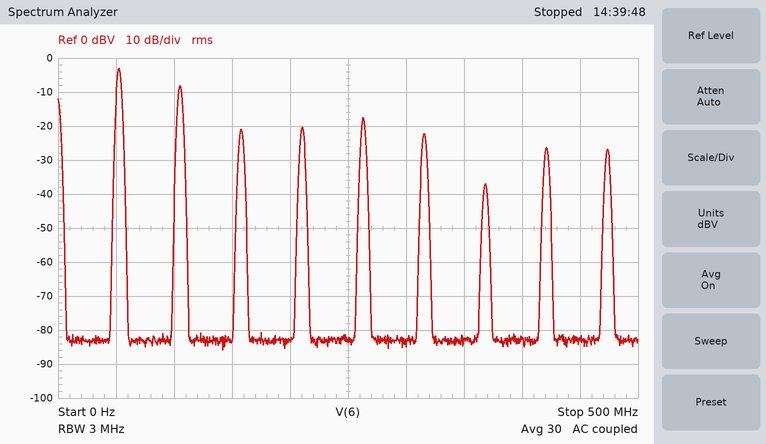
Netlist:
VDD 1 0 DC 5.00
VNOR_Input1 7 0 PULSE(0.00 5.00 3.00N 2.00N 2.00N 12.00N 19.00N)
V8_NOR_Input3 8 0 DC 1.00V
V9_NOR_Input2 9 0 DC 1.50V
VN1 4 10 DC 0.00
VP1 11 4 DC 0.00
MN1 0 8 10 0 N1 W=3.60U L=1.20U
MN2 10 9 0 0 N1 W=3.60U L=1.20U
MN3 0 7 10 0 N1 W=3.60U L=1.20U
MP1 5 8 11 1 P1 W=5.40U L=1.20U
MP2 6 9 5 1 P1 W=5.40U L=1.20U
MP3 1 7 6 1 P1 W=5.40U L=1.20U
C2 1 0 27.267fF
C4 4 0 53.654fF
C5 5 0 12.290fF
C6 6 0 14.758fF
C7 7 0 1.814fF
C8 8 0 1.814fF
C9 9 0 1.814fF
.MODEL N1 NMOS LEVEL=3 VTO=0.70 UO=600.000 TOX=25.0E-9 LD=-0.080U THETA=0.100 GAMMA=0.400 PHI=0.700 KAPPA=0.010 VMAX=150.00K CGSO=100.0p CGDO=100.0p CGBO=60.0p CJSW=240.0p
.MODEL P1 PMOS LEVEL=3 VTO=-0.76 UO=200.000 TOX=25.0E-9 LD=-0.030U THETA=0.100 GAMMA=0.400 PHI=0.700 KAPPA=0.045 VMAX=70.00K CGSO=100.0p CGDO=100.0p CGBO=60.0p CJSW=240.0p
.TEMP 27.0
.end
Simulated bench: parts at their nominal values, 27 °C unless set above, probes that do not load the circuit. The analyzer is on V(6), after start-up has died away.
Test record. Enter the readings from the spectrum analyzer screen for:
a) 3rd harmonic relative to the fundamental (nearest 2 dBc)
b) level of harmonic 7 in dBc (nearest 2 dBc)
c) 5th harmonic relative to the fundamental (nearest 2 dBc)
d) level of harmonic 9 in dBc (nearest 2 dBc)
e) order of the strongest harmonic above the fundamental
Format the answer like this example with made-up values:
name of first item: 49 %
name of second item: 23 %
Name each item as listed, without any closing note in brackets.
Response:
3rd harmonic relative to the fundamental: -18 dBc
level of harmonic 7 in dBc: -34 dBc
5th harmonic relative to the fundamental: -14 dBc
level of harmonic 9 in dBc: -24 dBc
order of the strongest harmonic above the fundamental: 2
